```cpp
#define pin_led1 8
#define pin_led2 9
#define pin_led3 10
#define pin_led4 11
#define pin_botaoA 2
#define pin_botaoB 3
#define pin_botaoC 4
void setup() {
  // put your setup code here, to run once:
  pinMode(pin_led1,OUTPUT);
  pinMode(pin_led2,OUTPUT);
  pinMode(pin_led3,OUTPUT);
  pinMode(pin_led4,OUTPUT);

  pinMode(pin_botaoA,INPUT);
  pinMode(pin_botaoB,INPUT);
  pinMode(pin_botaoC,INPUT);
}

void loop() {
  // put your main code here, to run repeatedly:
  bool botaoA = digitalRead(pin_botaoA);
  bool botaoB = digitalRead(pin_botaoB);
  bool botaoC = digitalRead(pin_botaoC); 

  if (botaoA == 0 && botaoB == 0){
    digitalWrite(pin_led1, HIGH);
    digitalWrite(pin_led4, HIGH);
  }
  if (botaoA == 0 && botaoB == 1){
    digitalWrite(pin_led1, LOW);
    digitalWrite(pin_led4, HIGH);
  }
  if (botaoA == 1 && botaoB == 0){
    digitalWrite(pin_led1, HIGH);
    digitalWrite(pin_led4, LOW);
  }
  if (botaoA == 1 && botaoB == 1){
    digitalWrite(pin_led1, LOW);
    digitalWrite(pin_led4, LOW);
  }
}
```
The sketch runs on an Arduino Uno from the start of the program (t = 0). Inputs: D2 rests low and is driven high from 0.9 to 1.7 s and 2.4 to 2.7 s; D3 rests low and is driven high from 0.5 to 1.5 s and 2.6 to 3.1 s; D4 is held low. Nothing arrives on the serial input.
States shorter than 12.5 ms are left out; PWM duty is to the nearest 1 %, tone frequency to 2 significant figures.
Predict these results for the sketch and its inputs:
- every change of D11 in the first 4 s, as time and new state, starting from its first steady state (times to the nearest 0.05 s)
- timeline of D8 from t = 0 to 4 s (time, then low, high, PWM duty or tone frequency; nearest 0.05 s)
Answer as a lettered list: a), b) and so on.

a) 0 s high; 0.9 s low; 1.7 s high; 2.4 s low; 2.7 s high
b) 0 s high; 0.5 s low; 1.5 s high; 2.6 s low; 3.1 s high
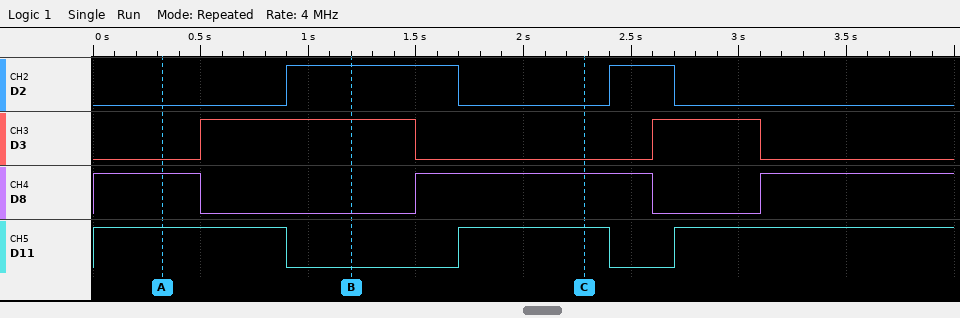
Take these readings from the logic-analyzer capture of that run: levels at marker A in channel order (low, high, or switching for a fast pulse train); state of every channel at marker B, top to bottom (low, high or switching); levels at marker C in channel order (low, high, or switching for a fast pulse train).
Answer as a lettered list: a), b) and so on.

a) D2 low, D3 low, D8 high, D11 high
b) D2 high, D3 high, D8 low, D11 low
c) D2 low, D3 low, D8 high, D11 high
